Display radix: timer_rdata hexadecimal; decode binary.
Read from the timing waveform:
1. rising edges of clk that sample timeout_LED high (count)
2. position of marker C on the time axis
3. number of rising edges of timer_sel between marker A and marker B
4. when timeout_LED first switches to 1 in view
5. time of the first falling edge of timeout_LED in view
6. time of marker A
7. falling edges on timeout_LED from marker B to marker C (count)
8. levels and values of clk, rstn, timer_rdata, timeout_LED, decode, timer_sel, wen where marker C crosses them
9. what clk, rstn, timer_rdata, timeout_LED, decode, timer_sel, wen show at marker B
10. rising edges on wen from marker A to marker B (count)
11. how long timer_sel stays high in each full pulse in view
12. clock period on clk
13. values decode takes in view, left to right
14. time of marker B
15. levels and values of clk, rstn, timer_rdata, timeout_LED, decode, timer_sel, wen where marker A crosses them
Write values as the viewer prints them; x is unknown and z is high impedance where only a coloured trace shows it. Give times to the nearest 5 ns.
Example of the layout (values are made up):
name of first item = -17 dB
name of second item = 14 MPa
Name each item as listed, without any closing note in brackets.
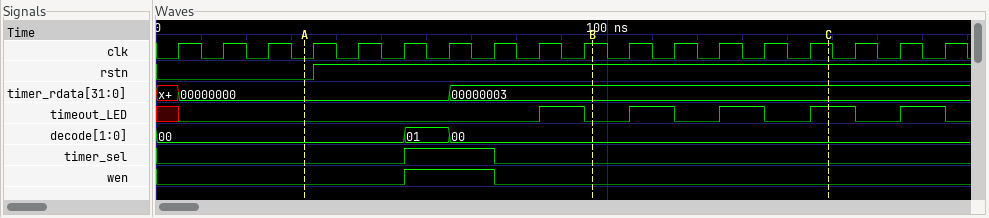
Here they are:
rising edges of clk that sample timeout_LED high = 5
position of marker C on the time axis = 150 ns
number of rising edges of timer_sel between marker A and marker B = 1
when timeout_LED first switches to 1 in view = 85 ns
time of the first falling edge of timeout_LED in view = 95 ns
time of marker A = 35 ns
falling edges on timeout_LED from marker B to marker C = 2
levels and values of clk, rstn, timer_rdata, timeout_LED, decode, timer_sel, wen where marker C crosses them = clk=1, rstn=1, timer_rdata=00000003, timeout_LED=1, decode=00, timer_sel=0, wen=0
what clk, rstn, timer_rdata, timeout_LED, decode, timer_sel, wen show at marker B = clk=1, rstn=1, timer_rdata=00000003, timeout_LED=0, decode=00, timer_sel=0, wen=0
rising edges on wen from marker A to marker B = 1
how long timer_sel stays high in each full pulse in view = 20 ns
clock period on clk = 10 ns
values decode takes in view, left to right = 00, 01, 00
time of marker B = 95 ns
levels and values of clk, rstn, timer_rdata, timeout_LED, decode, timer_sel, wen where marker A crosses them = clk=0, rstn=0, timer_rdata=00000000, timeout_LED=0, decode=00, timer_sel=0, wen=0
